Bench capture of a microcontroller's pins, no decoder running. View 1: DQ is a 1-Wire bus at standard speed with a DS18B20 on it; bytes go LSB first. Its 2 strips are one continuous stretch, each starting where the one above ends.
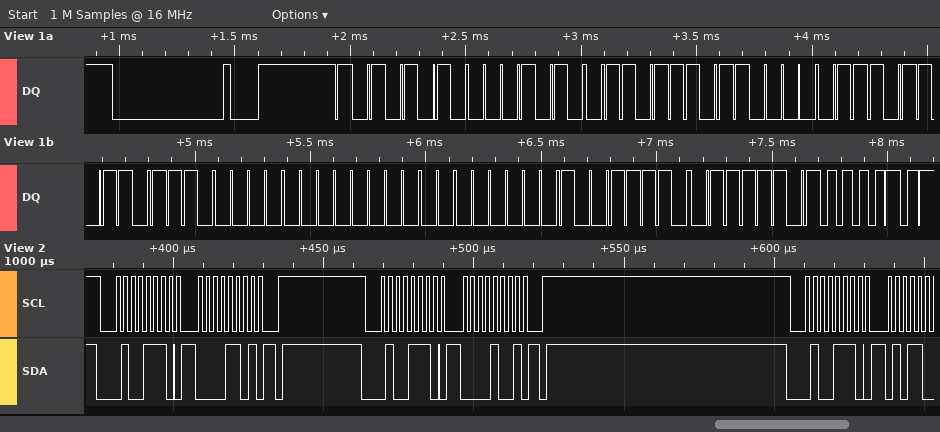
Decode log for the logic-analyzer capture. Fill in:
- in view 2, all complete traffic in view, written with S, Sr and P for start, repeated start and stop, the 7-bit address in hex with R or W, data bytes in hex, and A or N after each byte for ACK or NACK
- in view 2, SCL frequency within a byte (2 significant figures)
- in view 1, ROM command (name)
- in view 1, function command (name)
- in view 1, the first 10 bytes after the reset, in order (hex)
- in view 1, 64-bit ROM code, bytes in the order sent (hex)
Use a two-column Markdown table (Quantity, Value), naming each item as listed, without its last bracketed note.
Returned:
| Quantity | Value |
|---|---|
| in view 2, all complete traffic in view, written with S, Sr and P for start, repeated start and stop, the 7-bit address in hex with R or W, data bytes in hex, and A or N after each byte for ACK or NACK | S 27W A 0D A P S 27W A 09 A P S 27W A |
| in view 2, SCL frequency within a byte | 400 kHz |
| in view 1, ROM command | Match ROM |
| in view 1, function command | Read Scratchpad |
| in view 1, the first 10 bytes after the reset, in order | 55 28 BB C1 6D 07 00 00 79 BE |
| in view 1, 64-bit ROM code, bytes in the order sent | 28 BB C1 6D 07 00 00 79 |
